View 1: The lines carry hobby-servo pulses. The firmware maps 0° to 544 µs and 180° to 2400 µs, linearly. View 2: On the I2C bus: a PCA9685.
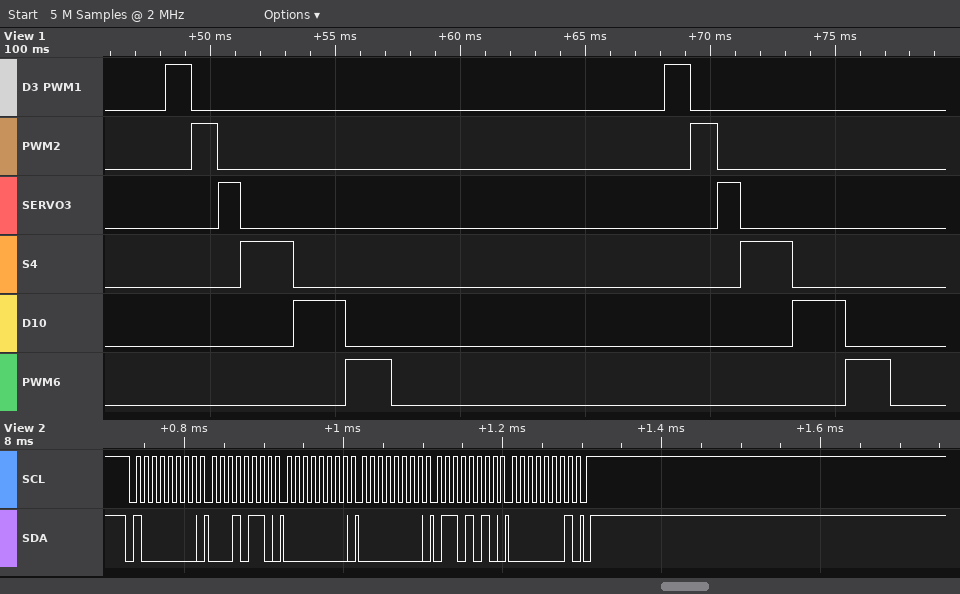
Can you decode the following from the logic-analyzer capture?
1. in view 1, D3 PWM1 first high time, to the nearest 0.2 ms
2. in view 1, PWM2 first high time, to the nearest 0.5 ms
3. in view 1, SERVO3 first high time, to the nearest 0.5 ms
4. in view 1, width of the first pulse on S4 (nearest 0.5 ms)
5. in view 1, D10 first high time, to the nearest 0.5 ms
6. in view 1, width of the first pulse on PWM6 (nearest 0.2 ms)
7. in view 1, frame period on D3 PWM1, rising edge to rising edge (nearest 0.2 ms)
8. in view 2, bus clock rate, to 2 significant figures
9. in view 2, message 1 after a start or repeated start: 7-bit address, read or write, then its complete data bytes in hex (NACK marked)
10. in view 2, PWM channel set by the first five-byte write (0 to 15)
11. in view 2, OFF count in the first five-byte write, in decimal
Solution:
1.0 ms
1.0 ms
1.0 ms
2.0 ms
2.0 ms
1.8 ms
20.0 ms
100 kHz
0x40 write: 16 00 00 6A 01
4
362
